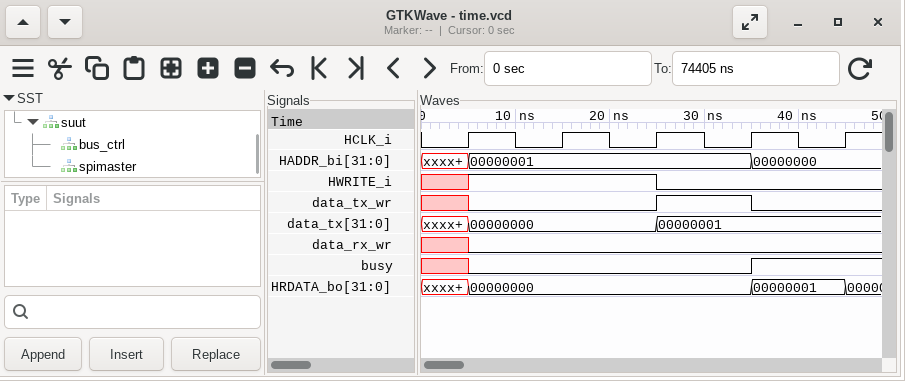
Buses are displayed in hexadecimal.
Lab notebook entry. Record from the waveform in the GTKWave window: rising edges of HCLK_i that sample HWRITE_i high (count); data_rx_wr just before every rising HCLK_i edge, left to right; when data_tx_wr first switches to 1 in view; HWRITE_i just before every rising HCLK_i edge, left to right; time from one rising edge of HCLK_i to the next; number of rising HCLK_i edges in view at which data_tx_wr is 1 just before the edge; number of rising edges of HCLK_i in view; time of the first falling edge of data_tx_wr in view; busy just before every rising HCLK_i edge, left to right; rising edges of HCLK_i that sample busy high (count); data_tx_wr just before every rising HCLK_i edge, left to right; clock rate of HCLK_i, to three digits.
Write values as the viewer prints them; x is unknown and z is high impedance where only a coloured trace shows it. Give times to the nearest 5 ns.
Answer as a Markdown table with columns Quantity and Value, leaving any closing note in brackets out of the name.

| Quantity | Value |
|---|---|
| rising edges of HCLK_i that sample HWRITE_i high | 2 |
| data_rx_wr just before every rising HCLK_i edge, left to right | x 0 0 0 0 |
| when data_tx_wr first switches to 1 in view | 25 ns |
| HWRITE_i just before every rising HCLK_i edge, left to right | x 1 1 0 0 |
| time from one rising edge of HCLK_i to the next | 10 ns |
| number of rising HCLK_i edges in view at which data_tx_wr is 1 just before the edge | 1 |
| number of rising edges of HCLK_i in view | 5 |
| time of the first falling edge of data_tx_wr in view | 35 ns |
| busy just before every rising HCLK_i edge, left to right | x 0 0 0 1 |
| rising edges of HCLK_i that sample busy high | 1 |
| data_tx_wr just before every rising HCLK_i edge, left to right | x 0 0 1 0 |
| clock rate of HCLK_i, to three digits | 100 MHz |
